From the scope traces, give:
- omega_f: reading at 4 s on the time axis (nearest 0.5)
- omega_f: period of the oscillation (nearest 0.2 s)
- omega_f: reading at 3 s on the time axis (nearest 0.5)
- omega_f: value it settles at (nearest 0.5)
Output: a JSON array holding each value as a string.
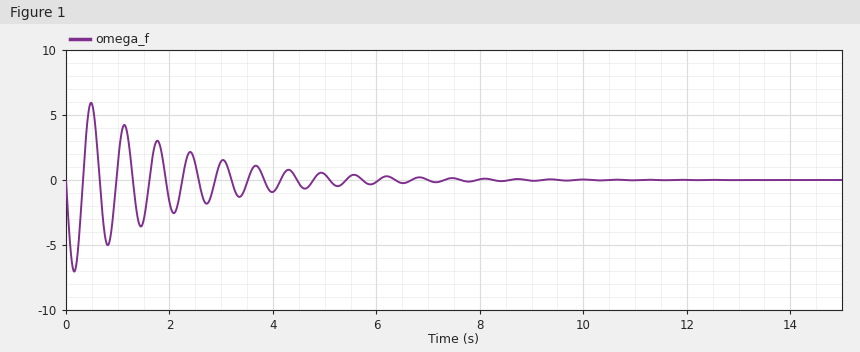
["-1.0", "0.6 s", "1.5", "0.0"]
